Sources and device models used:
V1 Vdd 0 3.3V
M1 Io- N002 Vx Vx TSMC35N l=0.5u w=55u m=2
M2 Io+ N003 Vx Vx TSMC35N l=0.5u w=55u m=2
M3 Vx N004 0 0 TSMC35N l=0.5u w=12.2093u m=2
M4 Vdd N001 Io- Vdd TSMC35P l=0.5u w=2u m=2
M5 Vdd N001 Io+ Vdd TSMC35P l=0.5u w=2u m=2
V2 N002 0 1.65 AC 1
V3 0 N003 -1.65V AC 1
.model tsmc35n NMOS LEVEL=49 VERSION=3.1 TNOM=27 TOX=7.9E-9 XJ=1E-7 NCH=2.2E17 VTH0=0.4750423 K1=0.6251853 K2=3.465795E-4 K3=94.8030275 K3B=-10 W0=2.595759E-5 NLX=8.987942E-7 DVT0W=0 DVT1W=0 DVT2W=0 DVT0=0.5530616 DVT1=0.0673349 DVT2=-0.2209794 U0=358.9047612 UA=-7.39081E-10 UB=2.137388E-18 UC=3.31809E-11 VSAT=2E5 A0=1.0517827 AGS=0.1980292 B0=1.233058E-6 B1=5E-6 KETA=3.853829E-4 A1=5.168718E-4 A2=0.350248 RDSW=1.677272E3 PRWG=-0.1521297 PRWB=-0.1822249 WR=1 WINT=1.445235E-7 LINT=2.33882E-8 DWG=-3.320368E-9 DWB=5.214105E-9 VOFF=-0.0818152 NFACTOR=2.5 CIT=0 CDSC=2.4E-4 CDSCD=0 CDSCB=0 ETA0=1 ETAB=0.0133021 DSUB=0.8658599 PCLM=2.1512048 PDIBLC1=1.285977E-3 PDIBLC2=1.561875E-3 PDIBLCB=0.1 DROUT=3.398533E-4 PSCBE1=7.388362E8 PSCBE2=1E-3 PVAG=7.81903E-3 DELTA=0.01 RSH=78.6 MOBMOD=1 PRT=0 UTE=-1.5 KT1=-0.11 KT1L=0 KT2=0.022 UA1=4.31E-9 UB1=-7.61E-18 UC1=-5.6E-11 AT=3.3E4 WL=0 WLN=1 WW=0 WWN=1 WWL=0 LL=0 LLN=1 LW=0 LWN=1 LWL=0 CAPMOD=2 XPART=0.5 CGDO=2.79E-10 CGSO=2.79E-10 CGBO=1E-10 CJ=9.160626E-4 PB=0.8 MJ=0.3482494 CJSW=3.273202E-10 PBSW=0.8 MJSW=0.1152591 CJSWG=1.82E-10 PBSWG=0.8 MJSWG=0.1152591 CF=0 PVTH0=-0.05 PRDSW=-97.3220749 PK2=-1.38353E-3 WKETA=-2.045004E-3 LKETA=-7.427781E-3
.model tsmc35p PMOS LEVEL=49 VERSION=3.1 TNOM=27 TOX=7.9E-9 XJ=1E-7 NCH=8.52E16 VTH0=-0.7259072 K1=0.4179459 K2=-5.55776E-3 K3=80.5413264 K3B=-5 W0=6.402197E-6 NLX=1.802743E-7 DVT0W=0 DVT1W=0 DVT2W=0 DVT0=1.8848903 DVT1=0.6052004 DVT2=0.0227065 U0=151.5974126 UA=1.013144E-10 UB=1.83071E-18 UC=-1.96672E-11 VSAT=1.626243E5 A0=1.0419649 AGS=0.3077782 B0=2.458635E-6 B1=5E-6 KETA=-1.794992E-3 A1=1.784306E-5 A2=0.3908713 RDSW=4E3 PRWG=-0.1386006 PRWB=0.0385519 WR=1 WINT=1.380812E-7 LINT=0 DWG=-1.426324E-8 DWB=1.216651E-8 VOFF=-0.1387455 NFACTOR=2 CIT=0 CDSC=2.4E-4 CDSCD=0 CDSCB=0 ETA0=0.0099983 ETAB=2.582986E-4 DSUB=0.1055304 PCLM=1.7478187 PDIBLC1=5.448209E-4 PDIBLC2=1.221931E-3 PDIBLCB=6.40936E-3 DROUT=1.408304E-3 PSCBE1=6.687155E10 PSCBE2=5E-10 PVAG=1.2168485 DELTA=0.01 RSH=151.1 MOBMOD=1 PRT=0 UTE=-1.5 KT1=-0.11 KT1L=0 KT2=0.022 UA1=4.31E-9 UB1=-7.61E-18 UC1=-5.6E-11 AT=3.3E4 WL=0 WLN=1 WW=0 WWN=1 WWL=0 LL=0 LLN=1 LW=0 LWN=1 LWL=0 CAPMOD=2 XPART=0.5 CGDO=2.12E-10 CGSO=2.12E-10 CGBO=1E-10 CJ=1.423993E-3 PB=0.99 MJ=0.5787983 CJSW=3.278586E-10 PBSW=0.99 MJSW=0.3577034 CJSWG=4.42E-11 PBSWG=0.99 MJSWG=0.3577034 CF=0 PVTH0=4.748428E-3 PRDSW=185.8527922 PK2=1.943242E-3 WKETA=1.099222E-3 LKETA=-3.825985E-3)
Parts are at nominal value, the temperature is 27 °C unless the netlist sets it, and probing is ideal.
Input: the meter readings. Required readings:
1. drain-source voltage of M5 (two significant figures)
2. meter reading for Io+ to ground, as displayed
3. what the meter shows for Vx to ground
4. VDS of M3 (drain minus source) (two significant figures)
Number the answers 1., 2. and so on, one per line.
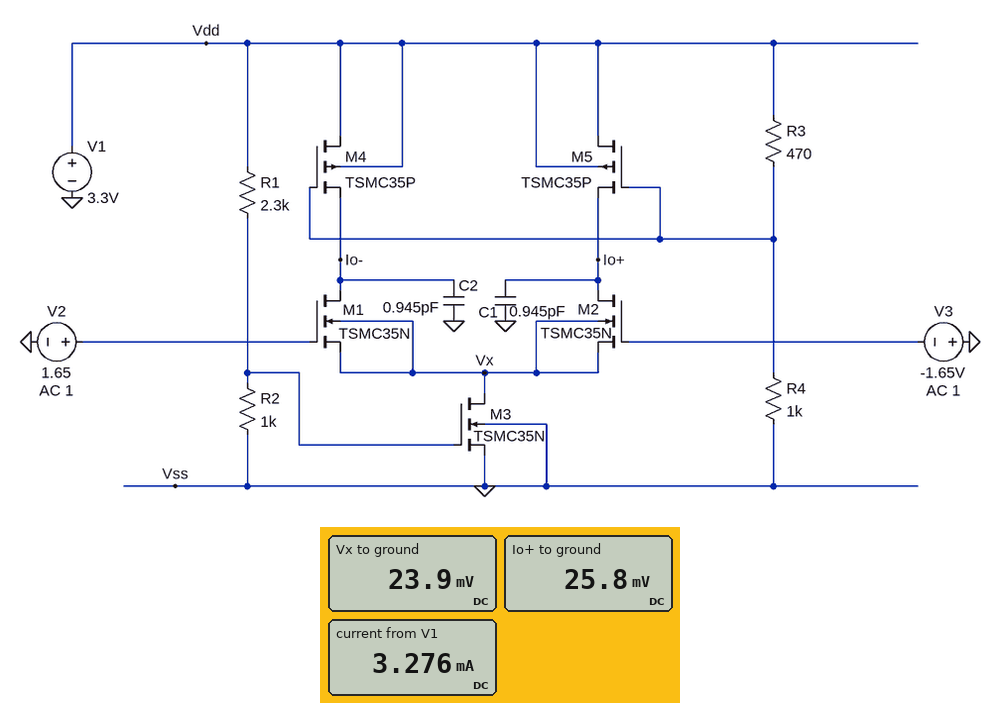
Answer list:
1. 3.3 V
2. 25.8 mV
3. 23.9 mV
4. 24 mV
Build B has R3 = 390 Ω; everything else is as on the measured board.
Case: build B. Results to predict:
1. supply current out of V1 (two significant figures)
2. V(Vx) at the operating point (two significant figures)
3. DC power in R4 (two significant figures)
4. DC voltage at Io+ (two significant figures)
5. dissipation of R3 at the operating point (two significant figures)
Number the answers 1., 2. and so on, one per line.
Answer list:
1. 3.4 mA
2. 8.2 mV
3. 5.6 mW
4. 8.9 mV
5. 2.2 mW
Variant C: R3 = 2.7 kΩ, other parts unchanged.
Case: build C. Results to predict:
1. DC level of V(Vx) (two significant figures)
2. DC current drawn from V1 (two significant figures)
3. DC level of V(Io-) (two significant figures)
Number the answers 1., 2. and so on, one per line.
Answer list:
1. 850 mV
2. 2.1 mA
3. 3.0 V
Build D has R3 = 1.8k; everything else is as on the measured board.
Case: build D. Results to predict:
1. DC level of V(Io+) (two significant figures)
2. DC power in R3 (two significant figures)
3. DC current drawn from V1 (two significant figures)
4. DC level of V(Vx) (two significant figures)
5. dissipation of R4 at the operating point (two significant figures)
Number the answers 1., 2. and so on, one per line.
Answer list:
1. 2.9 V
2. 2.5 mW
3. 2.4 mA
4. 850 mV
5. 1.4 mW
